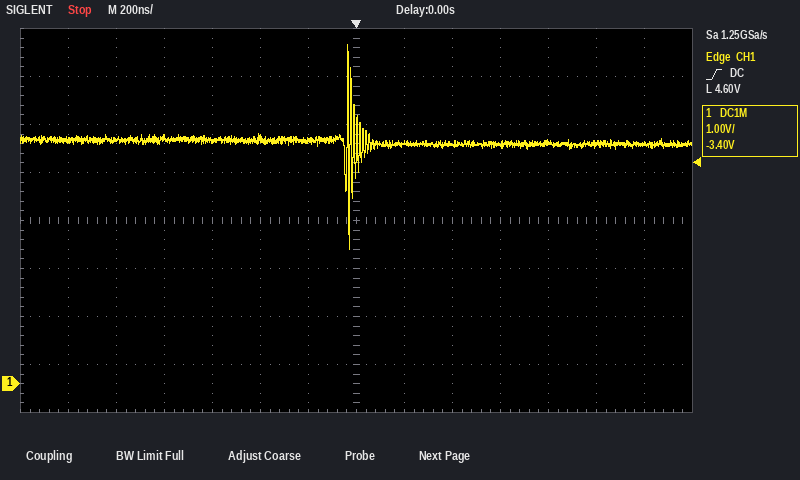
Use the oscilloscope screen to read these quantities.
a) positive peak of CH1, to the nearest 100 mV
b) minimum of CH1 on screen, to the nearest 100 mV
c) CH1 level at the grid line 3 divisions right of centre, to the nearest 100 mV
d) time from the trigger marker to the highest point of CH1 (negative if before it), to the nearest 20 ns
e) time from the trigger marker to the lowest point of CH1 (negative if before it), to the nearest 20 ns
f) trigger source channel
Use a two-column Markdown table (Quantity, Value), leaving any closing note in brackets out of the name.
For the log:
| Quantity | Value |
|---|---|
| positive peak of CH1, to the nearest 100 mV | 7.1 V |
| minimum of CH1 on screen, to the nearest 100 mV | 2.8 V |
| CH1 level at the grid line 3 divisions right of centre, to the nearest 100 mV | 5.0 V |
| time from the trigger marker to the highest point of CH1 (negative if before it), to the nearest 20 ns | -40 ns |
| time from the trigger marker to the lowest point of CH1 (negative if before it), to the nearest 20 ns | -20 ns |
| trigger source channel | CH1 |
